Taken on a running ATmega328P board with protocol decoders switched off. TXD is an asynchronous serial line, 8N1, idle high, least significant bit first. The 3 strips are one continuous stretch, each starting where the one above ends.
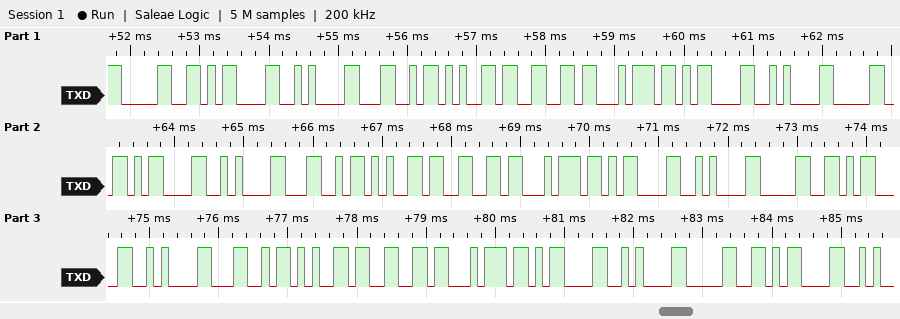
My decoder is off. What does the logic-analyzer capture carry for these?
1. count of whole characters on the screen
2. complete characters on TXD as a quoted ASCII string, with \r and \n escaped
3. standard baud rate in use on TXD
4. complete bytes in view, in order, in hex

29
"0\r\nLeft\r\n0\r\nLeft\r\n0\r\nLeft\r\n0\r"
9600 baud
30 0D 0A 4C 65 66 74 0D 0A 30 0D 0A 4C 65 66 74 0D 0A 30 0D 0A 4C 65 66 74 0D 0A 30 0D
